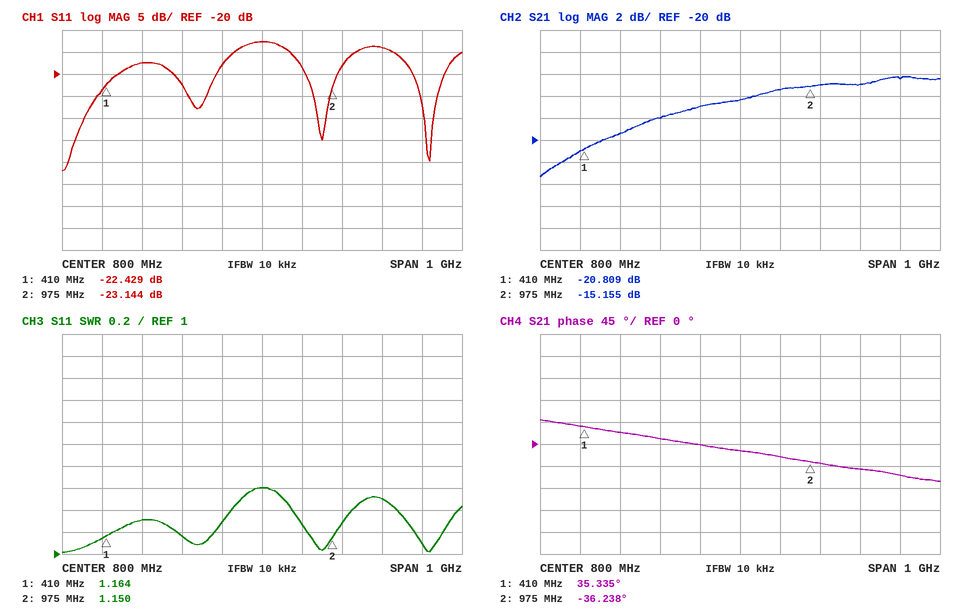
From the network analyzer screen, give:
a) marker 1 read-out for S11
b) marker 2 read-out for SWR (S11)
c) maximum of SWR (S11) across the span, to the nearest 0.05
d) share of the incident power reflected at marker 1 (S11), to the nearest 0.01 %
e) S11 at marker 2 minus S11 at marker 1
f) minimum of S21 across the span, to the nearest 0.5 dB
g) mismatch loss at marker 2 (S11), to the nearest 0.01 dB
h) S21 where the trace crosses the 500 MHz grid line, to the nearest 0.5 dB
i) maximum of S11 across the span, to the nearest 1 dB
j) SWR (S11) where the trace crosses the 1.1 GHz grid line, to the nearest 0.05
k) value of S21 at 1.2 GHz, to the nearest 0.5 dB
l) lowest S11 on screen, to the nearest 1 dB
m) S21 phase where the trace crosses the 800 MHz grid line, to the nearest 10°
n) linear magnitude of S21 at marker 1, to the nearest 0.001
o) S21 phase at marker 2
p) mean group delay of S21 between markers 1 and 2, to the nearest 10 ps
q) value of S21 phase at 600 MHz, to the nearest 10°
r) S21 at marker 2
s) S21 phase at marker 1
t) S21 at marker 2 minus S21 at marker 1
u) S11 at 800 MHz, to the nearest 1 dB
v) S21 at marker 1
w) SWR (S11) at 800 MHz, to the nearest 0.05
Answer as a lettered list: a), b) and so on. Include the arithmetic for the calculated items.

a) -22.429 dB
b) 1.150
c) 1.60
d) 10^(-22.429/10) ≈ 0.57 %
e) -23.144 − (-22.429) = -0.715 dB
f) -23.5 dB
g) −10 log10(1 − 10^(-23.144/10)) ≈ 0.02 dB
h) -19.5 dB
i) -13 dB
j) 1.50
k) -14.5 dB
l) -42 dB
m) -10°
n) 10^(-20.809/20) ≈ 0.091
o) -36.238°
p) −(-36.238° − (35.335°))/(360° × 565 MHz) ≈ 352 ps, so 350 ps to the nearest 10 ps
q) 10°
r) -15.155 dB
s) 35.335°
t) -15.155 − (-20.809) = 5.654 dB
u) -13 dB
v) -20.809 dB
w) 1.60
